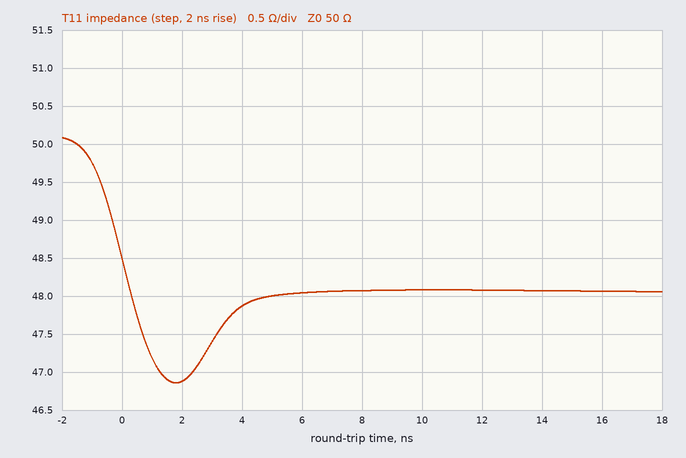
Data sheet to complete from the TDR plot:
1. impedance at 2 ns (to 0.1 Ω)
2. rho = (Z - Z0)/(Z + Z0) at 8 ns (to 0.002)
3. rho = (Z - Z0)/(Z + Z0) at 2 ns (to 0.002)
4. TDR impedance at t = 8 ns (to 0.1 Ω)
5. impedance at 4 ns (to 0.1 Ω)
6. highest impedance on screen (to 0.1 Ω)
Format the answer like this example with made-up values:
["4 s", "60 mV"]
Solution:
["46.9 Ω", "-0.020", "-0.032", "48.1 Ω", "47.9 Ω", "50.1 Ω"]
